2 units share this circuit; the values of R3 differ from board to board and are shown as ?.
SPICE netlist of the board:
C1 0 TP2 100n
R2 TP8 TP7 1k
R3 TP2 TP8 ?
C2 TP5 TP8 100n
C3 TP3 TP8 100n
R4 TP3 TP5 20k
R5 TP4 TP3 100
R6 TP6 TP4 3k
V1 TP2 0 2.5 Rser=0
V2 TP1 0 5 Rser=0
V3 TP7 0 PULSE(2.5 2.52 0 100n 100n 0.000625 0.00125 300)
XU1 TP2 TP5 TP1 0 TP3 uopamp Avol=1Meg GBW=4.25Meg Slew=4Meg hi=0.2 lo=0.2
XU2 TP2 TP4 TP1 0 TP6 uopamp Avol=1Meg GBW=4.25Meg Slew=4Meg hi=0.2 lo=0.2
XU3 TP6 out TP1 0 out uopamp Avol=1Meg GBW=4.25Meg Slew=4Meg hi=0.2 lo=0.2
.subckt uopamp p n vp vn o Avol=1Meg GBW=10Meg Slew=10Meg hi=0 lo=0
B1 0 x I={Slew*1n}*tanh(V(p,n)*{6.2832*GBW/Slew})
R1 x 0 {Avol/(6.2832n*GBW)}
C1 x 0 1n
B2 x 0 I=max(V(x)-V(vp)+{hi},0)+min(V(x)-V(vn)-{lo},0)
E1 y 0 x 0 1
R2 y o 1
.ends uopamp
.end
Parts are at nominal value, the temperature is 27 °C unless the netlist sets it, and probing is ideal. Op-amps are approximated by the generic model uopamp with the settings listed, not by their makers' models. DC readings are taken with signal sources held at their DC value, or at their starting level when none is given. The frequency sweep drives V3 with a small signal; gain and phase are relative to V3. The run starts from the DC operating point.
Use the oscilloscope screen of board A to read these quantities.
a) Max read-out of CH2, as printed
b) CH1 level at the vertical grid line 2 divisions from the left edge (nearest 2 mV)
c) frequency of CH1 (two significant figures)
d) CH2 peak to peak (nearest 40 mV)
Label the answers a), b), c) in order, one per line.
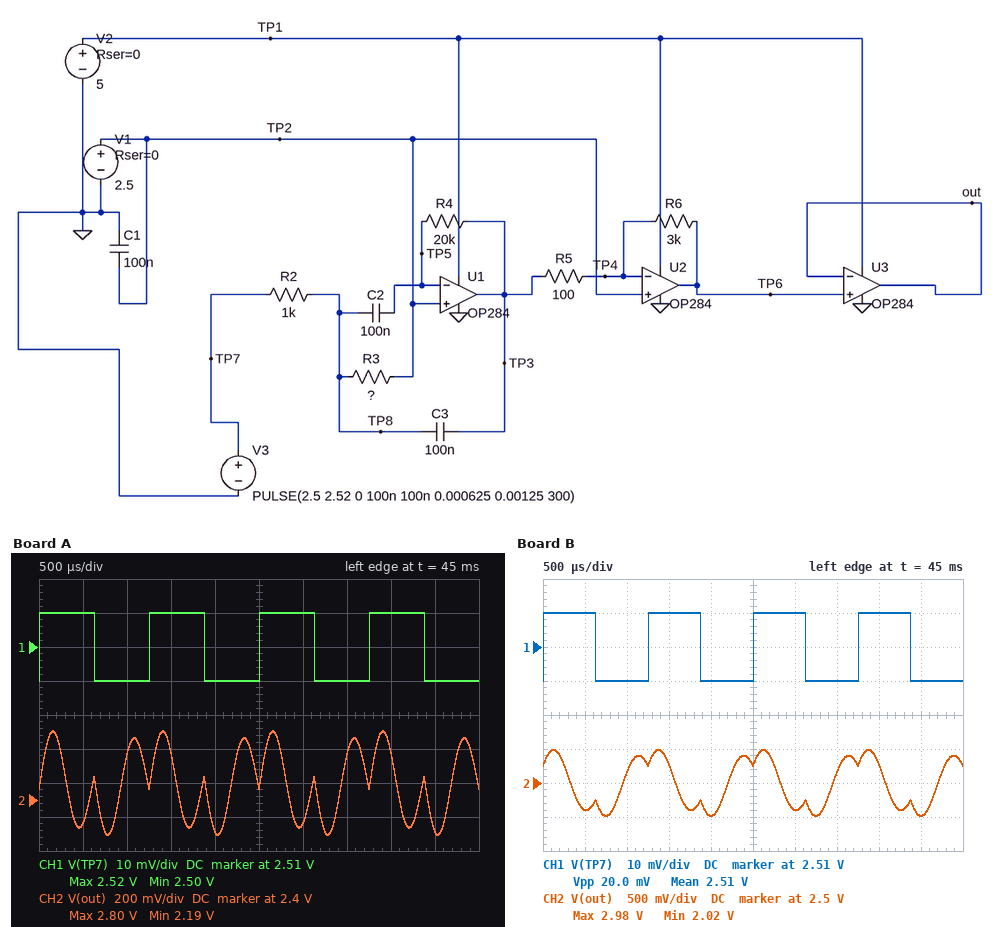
a) 2.80 V
b) 2.500 V
c) 800 Hz
d) 600 mV
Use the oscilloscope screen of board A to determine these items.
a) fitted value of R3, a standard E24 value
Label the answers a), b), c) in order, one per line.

a) 47 Ω
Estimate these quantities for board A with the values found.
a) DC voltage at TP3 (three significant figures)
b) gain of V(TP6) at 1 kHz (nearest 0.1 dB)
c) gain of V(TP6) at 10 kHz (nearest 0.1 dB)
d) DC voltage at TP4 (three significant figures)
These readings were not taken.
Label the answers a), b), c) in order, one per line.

a) 2.50 V
b) 28.4 dB
c) 13.7 dB
d) 2.50 V
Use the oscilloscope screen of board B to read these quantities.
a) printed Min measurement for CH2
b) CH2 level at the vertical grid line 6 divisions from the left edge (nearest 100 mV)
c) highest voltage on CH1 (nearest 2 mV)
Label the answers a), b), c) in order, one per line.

a) 2.02 V
b) 2.1 V
c) 2.520 V
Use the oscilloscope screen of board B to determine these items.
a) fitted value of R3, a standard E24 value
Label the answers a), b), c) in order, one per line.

a) 82 Ω
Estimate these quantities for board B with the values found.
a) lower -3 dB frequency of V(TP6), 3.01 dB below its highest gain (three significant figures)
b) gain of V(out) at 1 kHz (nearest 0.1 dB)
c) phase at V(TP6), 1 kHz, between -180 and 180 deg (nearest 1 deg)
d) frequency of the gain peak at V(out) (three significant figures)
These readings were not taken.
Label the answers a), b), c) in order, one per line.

a) 1.21 kHz
b) 36.9 dB
c) 76 deg
d) 1.29 kHz
